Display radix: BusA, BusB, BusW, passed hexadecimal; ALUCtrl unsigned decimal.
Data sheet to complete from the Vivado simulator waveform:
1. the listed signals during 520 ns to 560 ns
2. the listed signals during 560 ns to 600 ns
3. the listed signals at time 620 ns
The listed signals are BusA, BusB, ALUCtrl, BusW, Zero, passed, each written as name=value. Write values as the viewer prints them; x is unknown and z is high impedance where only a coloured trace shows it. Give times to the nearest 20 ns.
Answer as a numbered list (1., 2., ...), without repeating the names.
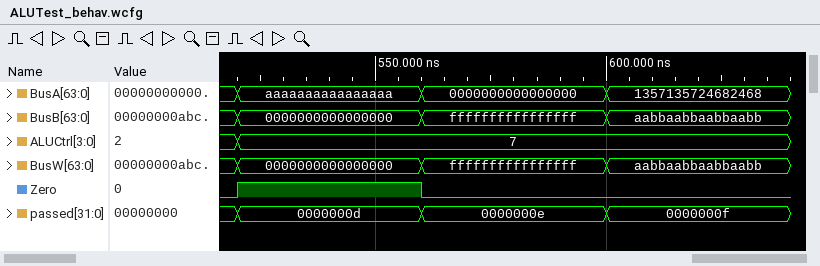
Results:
1. BusA=aaaaaaaaaaaaaaaa, BusB=0000000000000000, ALUCtrl=7, BusW=0000000000000000, Zero=1, passed=0000000d
2. BusA=0000000000000000, BusB=ffffffffffffffff, ALUCtrl=7, BusW=ffffffffffffffff, Zero=0, passed=0000000e
3. BusA=1357135724682468, BusB=aabbaabbaabbaabb, ALUCtrl=7, BusW=aabbaabbaabbaabb, Zero=0, passed=0000000f
